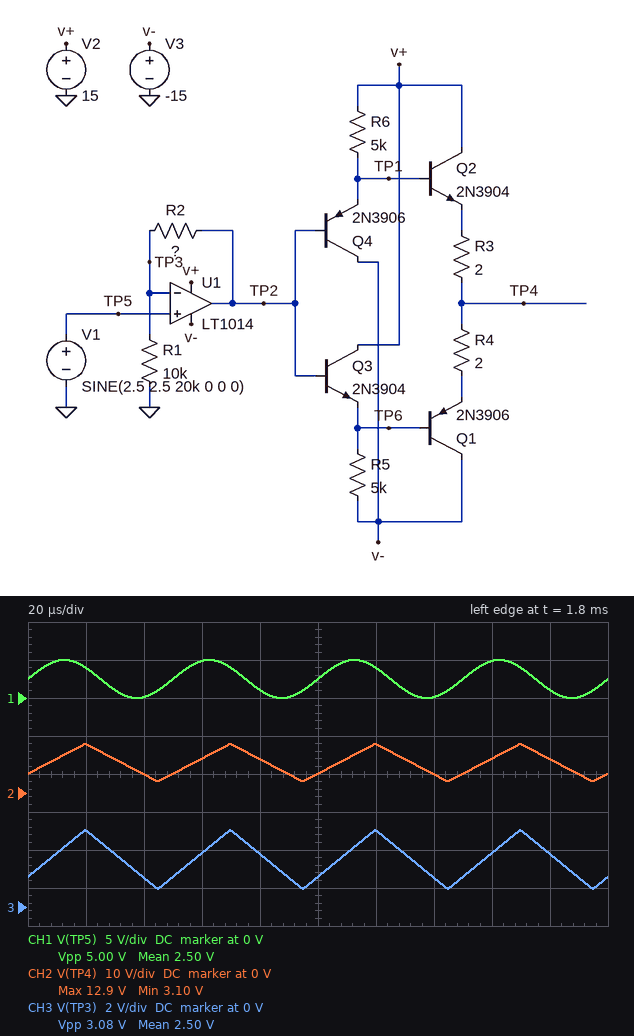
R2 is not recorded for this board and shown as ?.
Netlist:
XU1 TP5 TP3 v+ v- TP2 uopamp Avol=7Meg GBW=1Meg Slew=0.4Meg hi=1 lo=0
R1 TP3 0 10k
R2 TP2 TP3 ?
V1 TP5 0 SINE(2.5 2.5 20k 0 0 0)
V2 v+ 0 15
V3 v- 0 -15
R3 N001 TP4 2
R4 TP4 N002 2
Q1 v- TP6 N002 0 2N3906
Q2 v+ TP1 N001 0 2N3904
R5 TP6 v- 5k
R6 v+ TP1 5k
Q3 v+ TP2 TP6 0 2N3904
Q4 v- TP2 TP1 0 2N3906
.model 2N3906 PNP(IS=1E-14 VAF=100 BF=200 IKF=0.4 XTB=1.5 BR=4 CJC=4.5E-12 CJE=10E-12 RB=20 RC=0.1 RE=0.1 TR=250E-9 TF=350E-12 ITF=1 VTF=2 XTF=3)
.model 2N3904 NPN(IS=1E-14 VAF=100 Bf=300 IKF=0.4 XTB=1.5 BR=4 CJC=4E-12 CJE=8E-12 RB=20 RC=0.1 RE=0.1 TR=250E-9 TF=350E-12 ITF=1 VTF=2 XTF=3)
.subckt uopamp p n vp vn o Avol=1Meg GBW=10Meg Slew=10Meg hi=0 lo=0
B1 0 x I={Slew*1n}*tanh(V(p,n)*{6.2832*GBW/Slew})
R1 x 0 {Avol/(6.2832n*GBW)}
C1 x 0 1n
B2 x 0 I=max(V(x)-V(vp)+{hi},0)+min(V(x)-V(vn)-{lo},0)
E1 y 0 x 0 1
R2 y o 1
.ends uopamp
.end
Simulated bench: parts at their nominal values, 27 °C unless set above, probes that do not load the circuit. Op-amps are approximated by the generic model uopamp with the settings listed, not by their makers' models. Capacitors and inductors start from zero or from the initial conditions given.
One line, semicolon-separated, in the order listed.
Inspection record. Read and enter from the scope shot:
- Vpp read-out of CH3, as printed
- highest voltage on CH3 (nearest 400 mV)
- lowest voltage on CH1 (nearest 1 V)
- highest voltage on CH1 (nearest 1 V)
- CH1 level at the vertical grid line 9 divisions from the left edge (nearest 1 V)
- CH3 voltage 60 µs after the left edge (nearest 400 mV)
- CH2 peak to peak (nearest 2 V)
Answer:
3.08 V; 4.0 V; 0 V; 5 V; 1 V; 2.8 V; 10 V
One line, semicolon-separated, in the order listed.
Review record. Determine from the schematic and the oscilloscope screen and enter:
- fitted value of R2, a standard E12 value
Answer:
22 kΩ
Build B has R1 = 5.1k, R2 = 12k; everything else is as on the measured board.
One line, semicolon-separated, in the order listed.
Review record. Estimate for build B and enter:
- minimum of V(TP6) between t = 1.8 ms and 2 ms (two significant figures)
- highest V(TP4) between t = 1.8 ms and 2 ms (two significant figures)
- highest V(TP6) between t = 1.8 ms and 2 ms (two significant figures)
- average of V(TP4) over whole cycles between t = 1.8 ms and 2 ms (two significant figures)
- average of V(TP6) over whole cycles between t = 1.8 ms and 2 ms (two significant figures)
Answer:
2.8 V; 13 V; 13 V; 8.4 V; 7.7 V
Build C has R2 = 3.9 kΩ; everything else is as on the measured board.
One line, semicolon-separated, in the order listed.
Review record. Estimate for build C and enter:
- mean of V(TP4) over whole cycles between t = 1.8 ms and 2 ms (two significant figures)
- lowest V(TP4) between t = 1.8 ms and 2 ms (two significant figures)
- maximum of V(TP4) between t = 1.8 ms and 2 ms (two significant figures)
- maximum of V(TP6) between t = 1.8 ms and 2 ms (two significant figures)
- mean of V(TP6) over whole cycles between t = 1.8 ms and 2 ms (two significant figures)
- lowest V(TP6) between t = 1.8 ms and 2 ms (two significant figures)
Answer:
3.5 V; 1.4 mV; 6.9 V; 6.3 V; 2.8 V; -680 mV
